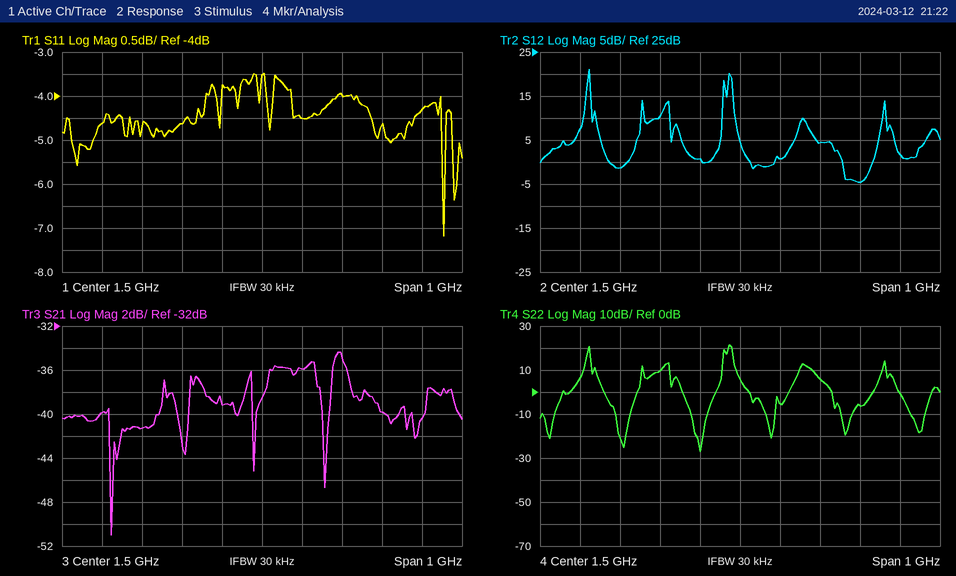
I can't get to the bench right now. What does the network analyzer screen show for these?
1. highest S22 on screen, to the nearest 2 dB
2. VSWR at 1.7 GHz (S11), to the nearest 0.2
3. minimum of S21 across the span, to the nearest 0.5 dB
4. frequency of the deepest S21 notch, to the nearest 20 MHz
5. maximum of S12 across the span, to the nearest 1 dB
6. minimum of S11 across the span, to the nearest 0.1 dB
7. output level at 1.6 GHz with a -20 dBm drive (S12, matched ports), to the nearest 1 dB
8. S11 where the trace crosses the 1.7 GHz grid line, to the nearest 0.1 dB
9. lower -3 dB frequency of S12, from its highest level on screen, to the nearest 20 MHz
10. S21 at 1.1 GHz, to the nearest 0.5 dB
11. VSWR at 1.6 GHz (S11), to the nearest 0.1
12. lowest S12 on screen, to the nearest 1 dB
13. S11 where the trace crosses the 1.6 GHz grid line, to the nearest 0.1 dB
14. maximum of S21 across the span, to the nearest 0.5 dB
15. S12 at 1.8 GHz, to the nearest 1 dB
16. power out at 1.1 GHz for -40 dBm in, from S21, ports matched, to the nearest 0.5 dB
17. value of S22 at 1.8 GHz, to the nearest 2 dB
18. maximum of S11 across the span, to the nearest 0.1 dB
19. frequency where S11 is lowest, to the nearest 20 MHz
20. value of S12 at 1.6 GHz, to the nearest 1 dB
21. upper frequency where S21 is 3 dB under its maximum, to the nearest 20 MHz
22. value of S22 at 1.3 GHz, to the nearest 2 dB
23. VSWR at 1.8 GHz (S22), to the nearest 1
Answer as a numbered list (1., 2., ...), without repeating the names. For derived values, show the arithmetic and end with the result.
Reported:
1. 22 dB
2. |Γ| = 10^(-4/20) = 0.6310; VSWR = (1 + 0.6310)/(1 − 0.6310) ≈ 4.4
3. -51.0 dB
4. 1.12 GHz
5. 21 dB
6. -7.2 dB
7. -20 dBm + (1 dB) = -19 dBm
8. -4.0 dB
9. 1.12 GHz
10. -40.0 dB
11. |Γ| = 10^(-4.5/20) = 0.5957; VSWR = (1 + 0.5957)/(1 − 0.5957) ≈ 3.9
12. -5 dB
13. -4.5 dB
14. -34.5 dB
15. -5 dB
16. -40 dBm + (-40.0 dB) = -80.0 dBm
17. -6 dB
18. -3.5 dB
19. 1.96 GHz
20. 1 dB
21. 1.72 GHz
22. 10 dB
23. |Γ| = 10^(-6/20) = 0.5012; VSWR = (1 + 0.5012)/(1 − 0.5012) ≈ 3
